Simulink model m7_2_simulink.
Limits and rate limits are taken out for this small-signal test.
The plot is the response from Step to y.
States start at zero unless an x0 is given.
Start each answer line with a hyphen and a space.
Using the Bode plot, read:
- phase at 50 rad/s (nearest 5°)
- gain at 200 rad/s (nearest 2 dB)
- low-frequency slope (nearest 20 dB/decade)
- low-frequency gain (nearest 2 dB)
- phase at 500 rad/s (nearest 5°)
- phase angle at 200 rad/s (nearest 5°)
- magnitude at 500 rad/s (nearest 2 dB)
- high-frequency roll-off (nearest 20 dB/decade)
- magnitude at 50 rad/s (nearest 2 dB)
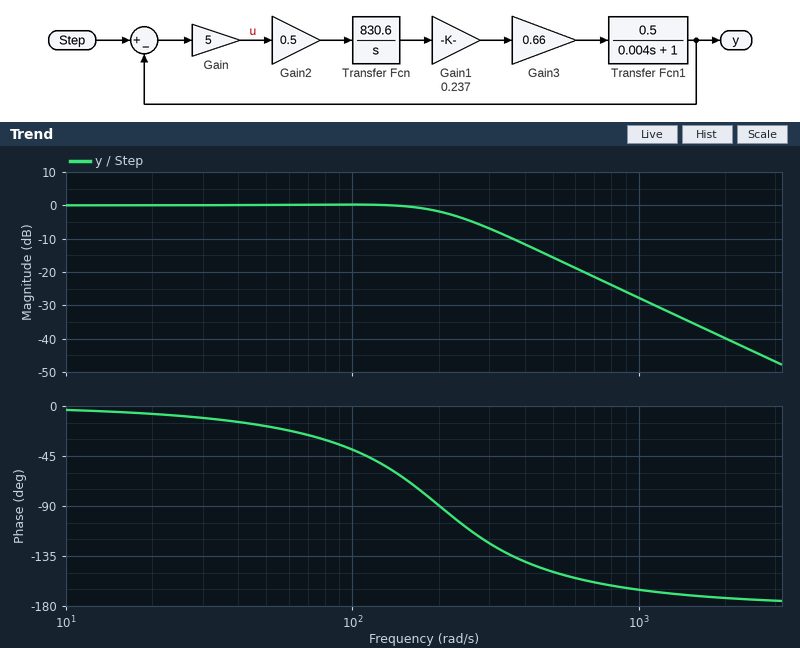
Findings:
- -20°
- -2 dB
- 0 dB/decade
- 0 dB
- -150°
- -90°
- -16 dB
- -40 dB/decade
- 0 dB
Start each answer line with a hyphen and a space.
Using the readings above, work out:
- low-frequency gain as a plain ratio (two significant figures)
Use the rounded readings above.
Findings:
- 1.0
